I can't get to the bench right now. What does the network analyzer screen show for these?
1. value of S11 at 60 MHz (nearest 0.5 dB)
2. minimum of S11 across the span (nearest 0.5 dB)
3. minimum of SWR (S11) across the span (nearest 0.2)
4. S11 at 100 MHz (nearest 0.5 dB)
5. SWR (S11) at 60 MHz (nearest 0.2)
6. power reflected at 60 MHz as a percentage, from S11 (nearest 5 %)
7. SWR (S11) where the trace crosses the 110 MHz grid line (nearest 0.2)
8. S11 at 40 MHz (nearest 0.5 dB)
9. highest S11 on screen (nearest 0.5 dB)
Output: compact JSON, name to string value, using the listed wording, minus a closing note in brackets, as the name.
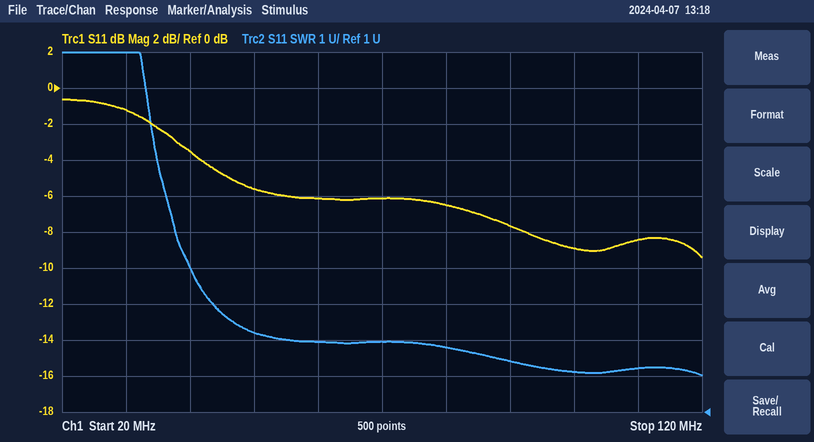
{"value of S11 at 60 MHz": "-6.0 dB", "minimum of S11 across the span": "-9.5 dB", "minimum of SWR (S11) across the span": "2.0", "S11 at 100 MHz": "-9.0 dB", "SWR (S11) at 60 MHz": "3.0", "power reflected at 60 MHz as a percentage, from S11": "25 %", "SWR (S11) where the trace crosses the 110 MHz grid line": "2.2", "S11 at 40 MHz": "-3.5 dB", "highest S11 on screen": "-0.5 dB"}
